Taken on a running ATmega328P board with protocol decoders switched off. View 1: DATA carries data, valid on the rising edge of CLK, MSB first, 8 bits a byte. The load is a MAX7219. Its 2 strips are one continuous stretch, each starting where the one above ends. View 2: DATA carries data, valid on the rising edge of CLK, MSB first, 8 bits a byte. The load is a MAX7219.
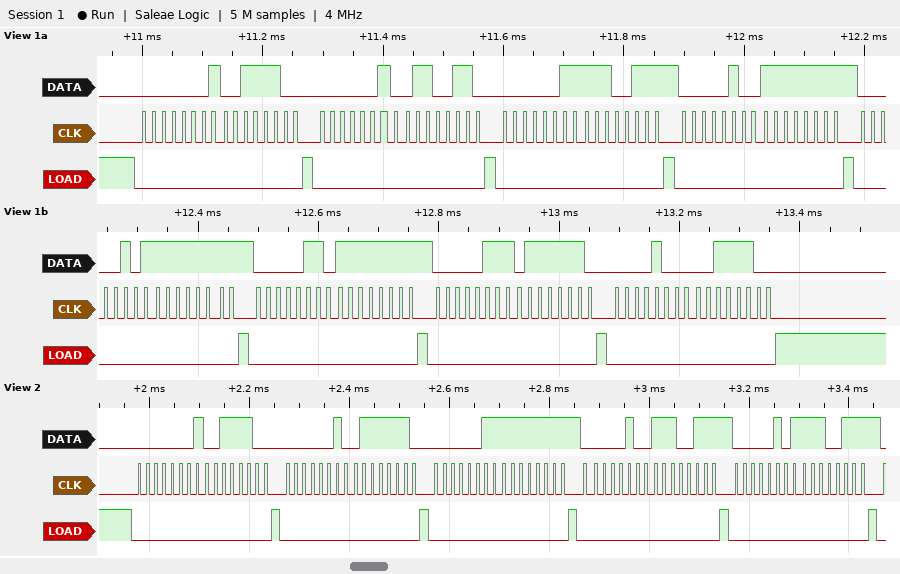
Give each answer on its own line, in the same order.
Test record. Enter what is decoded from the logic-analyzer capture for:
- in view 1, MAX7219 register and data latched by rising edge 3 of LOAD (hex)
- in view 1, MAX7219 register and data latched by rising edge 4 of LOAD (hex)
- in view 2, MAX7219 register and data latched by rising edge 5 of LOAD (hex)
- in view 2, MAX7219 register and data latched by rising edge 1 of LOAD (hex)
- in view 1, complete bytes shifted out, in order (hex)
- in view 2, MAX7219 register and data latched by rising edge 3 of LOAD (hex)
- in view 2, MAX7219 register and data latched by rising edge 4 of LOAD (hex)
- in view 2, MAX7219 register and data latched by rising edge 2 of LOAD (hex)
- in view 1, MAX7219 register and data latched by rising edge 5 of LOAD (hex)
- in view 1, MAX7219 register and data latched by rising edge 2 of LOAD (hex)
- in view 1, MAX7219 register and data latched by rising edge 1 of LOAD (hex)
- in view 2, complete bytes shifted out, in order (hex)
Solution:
register 0x3, data 0xE7
register 0x4, data 0xFF
register 0x5, data 0xE7
register 0x1, data 0x3C
01 3C 02 66 03 E7 04 FF 05 FF 06 FF 07 7E 08 3C
register 0x3, data 0xFF
register 0x4, data 0xE7
register 0x2, data 0x7E
register 0x5, data 0xFF
register 0x2, data 0x66
register 0x1, data 0x3C
01 3C 02 7E 03 FF 04 E7 05 E7
